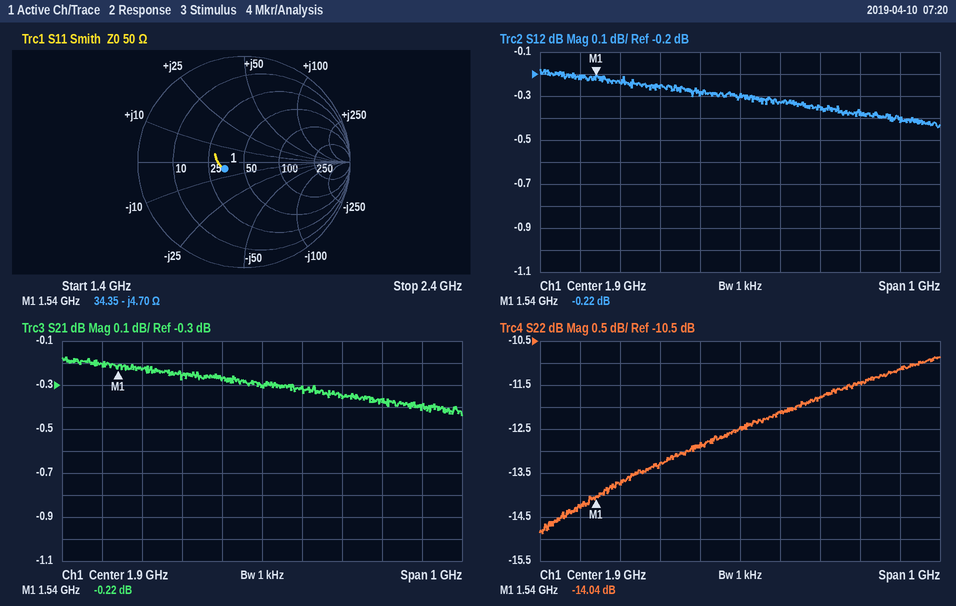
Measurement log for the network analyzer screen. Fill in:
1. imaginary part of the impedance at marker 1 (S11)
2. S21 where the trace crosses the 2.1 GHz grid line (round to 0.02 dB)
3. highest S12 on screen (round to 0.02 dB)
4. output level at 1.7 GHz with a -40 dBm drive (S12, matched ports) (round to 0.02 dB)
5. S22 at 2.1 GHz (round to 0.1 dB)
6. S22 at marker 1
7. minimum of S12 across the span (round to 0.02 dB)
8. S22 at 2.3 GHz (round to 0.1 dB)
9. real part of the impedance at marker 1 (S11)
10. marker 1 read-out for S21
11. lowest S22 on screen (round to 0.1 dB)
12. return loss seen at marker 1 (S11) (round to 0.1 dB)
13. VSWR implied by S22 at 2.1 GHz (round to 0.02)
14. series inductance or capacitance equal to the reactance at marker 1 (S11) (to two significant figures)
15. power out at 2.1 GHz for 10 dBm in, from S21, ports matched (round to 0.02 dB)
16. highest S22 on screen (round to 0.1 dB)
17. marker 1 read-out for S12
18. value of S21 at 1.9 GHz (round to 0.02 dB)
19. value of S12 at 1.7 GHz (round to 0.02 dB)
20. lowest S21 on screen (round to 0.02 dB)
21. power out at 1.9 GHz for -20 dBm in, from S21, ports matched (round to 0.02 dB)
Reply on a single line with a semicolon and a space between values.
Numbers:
-4.70 Ω; -0.36 dB; -0.18 dB; -40.26 dBm; -11.8 dB; -14.04 dB; -0.44 dB; -11.1 dB; 34.35 Ω; -0.22 dB; -14.9 dB; 14.3 dB; 1.70; 22 pF; 9.64 dBm; -10.9 dB; -0.22 dB; -0.30 dB; -0.26 dB; -0.44 dB; -20.30 dBm
